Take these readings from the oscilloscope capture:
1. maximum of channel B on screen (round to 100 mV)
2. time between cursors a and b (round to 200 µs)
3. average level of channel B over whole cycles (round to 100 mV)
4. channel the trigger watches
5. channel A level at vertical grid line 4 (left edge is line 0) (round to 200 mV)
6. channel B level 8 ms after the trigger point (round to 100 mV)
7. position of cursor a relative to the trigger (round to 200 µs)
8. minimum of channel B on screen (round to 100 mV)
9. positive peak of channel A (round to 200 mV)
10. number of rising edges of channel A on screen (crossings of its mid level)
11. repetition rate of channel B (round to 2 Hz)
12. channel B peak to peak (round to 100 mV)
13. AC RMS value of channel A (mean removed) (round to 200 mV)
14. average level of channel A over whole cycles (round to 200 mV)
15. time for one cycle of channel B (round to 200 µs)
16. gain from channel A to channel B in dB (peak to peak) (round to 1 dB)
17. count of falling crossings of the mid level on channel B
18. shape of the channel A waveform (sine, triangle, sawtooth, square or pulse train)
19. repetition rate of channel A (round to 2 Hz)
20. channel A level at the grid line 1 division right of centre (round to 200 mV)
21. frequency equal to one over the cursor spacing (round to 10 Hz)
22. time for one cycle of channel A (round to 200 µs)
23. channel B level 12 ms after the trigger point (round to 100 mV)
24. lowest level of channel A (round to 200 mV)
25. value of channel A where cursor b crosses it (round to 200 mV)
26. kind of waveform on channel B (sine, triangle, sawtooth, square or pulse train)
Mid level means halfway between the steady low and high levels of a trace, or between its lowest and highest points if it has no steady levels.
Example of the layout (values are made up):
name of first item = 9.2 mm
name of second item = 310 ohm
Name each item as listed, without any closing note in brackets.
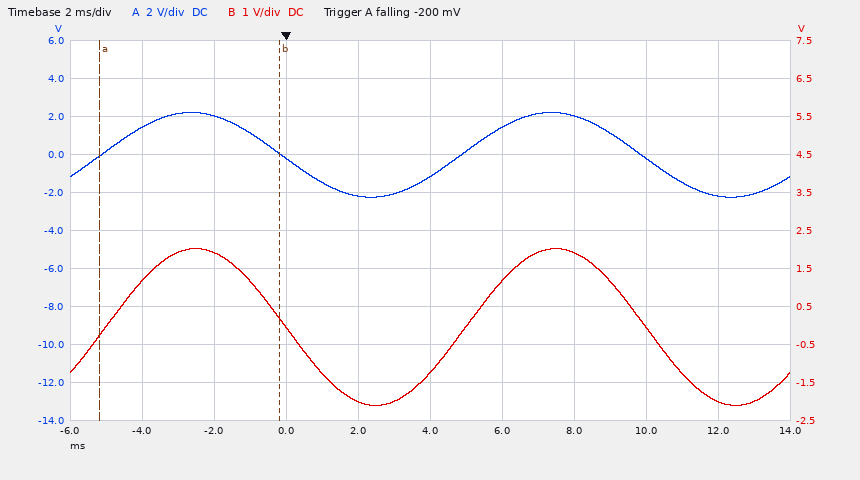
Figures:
maximum of channel B on screen = 2.0 V
time between cursors a and b = 5.0 ms
average level of channel B over whole cycles = 0.0 V
channel the trigger watches = channel A
channel A level at vertical grid line 4 (left edge is line 0) = -2.2 V
channel B level 8 ms after the trigger point = 1.9 V
position of cursor a relative to the trigger = -5.2 ms
minimum of channel B on screen = -2.1 V
positive peak of channel A = 2.2 V
number of rising edges of channel A on screen = 2
repetition rate of channel B = 100 Hz
channel B peak to peak = 4.1 V
AC RMS value of channel A (mean removed) = 1.6 V
average level of channel A over whole cycles = 0.0 V
time for one cycle of channel B = 10.0 ms
gain from channel A to channel B in dB (peak to peak) = -1 dB
count of falling crossings of the mid level on channel B = 2
shape of the channel A waveform = sine
repetition rate of channel A = 100 Hz
channel A level at the grid line 1 division right of centre = 1.4 V
frequency equal to one over the cursor spacing = 200 Hz
time for one cycle of channel A = 10.0 ms
channel B level 12 ms after the trigger point = -2.0 V
lowest level of channel A = -2.2 V
value of channel A where cursor b crosses it = 0.0 V
kind of waveform on channel B = sine
